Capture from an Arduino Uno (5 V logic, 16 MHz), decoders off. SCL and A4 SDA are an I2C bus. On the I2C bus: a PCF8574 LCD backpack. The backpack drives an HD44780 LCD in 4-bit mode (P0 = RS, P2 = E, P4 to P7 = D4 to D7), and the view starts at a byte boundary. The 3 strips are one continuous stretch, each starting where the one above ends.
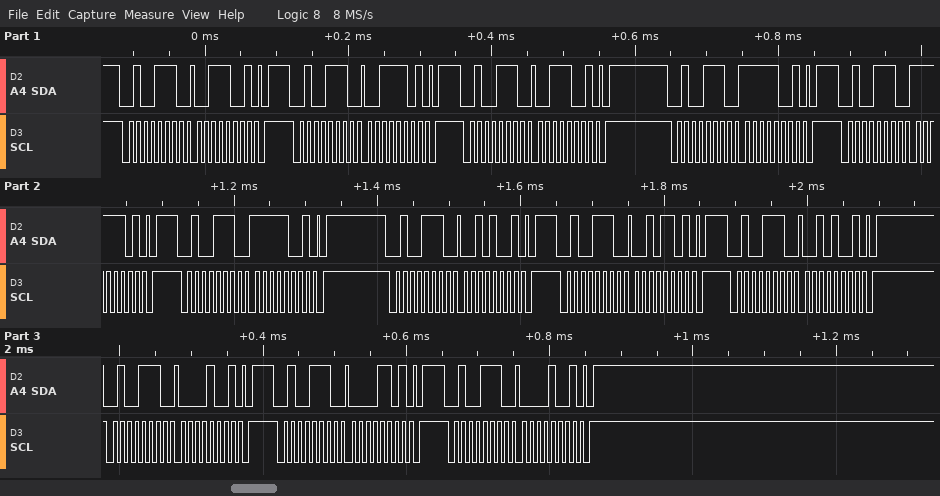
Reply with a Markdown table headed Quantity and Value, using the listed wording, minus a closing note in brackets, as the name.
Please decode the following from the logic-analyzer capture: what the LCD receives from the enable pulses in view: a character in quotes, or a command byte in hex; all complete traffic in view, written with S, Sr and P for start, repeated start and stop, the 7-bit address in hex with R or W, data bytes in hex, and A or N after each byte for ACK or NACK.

| Quantity | Value |
|---|---|
| what the LCD receives from the enable pulses in view: a character in quotes, or a command byte in hex | '?' ' ' |
| all complete traffic in view, written with S, Sr and P for start, repeated start and stop, the 7-bit address in hex with R or W, data bytes in hex, and A or N after each byte for ACK or NACK | S 27W A 39 A P S 27W A 3D A P S 27W A 39 A P S 27W A F9 A P S 27W A FD A P S 27W A F9 A P S 27W A 29 A P S 27W A 2D A P S 27W A 29 A P S 27W A 09 A P S 27W A 0D A P S 27W A 09 A P |
